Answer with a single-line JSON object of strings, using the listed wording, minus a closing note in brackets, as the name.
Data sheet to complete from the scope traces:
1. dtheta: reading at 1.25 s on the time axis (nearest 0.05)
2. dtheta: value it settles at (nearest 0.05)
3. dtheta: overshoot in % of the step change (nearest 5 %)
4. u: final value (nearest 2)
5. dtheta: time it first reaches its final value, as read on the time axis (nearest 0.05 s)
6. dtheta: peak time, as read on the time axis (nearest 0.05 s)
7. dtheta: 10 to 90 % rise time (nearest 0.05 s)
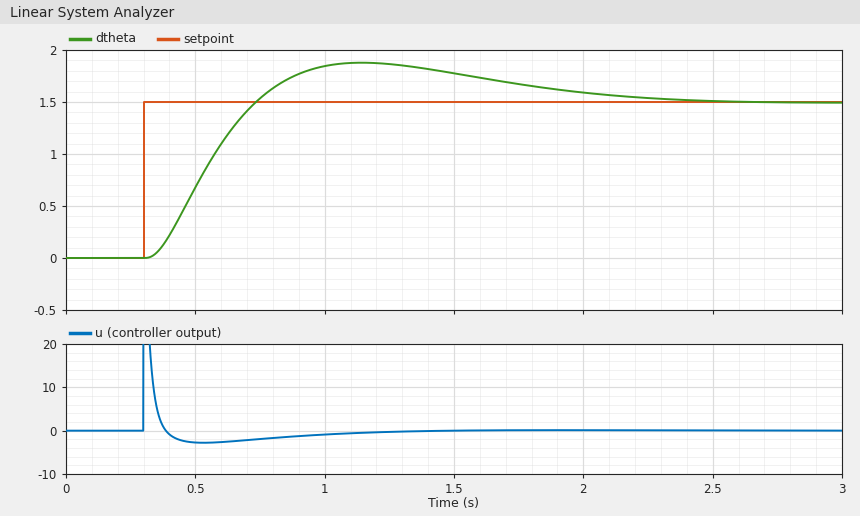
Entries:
{"dtheta: reading at 1.25 s on the time axis": "1.85", "dtheta: value it settles at": "1.50", "dtheta: overshoot in % of the step change": "25 %", "u: final value": "0", "dtheta: time it first reaches its final value, as read on the time axis": "0.75 s", "dtheta: peak time, as read on the time axis": "1.15 s", "dtheta: 10 to 90 % rise time": "0.30 s"}
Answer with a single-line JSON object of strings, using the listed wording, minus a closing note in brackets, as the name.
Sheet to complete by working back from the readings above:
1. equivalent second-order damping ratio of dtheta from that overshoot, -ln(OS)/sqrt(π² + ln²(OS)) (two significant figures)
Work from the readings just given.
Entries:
{"equivalent second-order damping ratio of dtheta from that overshoot, -ln(OS)/sqrt(π² + ln²(OS))": "0.40"}
